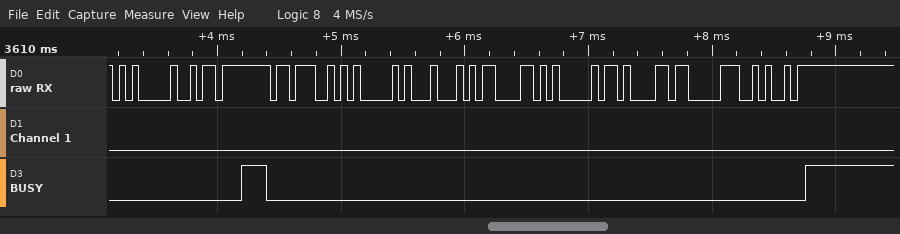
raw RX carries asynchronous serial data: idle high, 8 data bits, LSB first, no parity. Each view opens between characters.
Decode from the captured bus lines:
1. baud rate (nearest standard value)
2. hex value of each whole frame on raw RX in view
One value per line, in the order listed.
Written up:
19200 baud
05, DA, 3B, 05, 11, 0D, 05, 0B, 83, 4A
